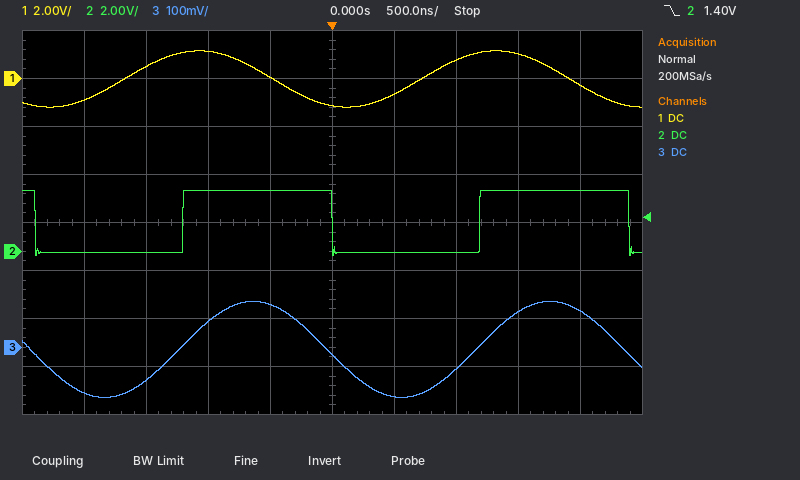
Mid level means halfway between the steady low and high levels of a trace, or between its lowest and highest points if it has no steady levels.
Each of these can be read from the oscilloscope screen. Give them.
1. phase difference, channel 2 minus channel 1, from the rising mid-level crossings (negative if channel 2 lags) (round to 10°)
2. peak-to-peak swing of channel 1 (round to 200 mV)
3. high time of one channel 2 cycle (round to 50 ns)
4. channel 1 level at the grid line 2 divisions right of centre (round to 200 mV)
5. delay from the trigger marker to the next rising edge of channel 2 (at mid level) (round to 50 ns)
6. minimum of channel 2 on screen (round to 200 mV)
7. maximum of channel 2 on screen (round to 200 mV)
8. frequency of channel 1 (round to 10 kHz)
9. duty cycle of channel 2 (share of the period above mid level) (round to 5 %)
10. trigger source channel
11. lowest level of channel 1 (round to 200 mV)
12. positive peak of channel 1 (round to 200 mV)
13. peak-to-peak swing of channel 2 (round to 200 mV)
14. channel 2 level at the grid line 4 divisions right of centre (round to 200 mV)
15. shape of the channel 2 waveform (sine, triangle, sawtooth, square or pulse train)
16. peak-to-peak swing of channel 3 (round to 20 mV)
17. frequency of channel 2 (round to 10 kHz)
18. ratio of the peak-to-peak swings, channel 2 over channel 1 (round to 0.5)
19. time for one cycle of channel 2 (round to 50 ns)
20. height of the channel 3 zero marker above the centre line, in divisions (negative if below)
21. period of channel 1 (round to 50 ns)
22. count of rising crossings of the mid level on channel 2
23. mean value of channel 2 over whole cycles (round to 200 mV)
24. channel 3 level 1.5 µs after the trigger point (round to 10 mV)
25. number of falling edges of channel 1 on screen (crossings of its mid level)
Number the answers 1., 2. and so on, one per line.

1. -70°
2. 2.4 V
3. 1.20 µs
4. 800 mV
5. 1.20 µs
6. -200 mV
7. 2.6 V
8. 420 kHz
9. 50 %
10. channel 2
11. -1.2 V
12. 1.2 V
13. 2.8 V
14. 2.6 V
15. square
16. 200 mV
17. 420 kHz
18. 1.0
19. 2.40 µs
20. -2.6 div
21. 2.40 µs
22. 2
23. 1.2 V
24. 70 mV
25. 2
